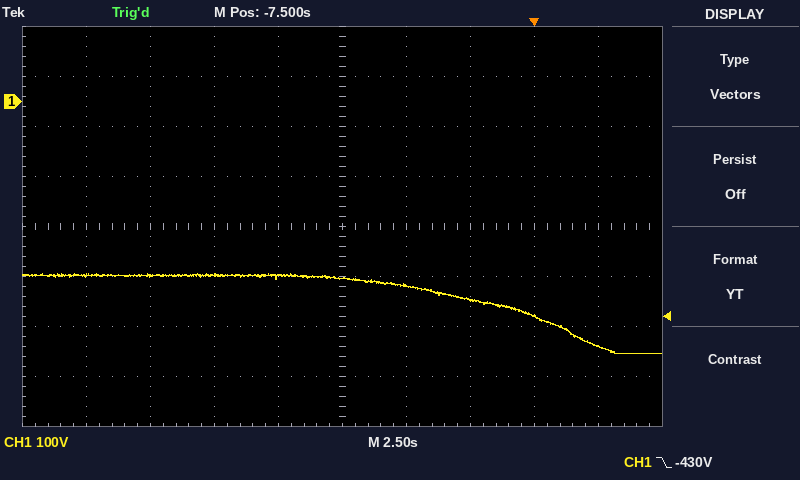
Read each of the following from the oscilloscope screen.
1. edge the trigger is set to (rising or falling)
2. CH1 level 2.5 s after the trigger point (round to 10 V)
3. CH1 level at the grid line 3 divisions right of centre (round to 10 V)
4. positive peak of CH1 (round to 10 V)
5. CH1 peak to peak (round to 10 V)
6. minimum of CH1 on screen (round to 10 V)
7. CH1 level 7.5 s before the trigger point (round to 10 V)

falling
-490 V
-430 V
-340 V
160 V
-500 V
-350 V
